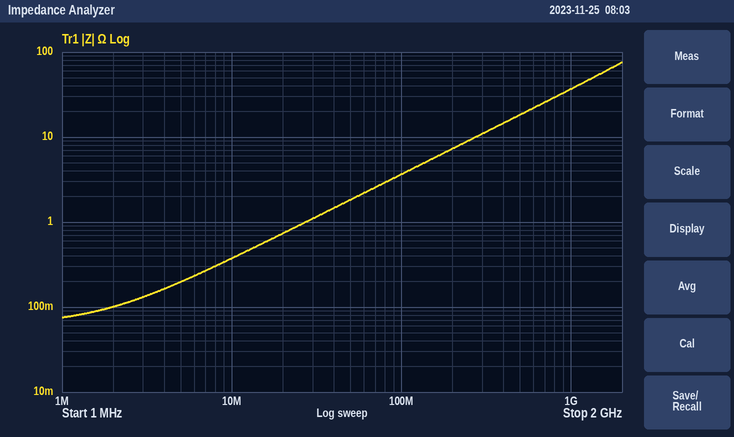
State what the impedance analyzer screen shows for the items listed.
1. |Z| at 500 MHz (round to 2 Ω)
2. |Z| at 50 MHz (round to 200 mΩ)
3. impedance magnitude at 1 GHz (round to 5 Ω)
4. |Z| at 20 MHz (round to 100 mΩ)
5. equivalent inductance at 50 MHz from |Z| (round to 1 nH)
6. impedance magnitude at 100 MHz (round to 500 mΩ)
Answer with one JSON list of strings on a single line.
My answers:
["18 Ω", "1.8 Ω", "35 Ω", "700 mΩ", "6 nH", "3.5 Ω"]
